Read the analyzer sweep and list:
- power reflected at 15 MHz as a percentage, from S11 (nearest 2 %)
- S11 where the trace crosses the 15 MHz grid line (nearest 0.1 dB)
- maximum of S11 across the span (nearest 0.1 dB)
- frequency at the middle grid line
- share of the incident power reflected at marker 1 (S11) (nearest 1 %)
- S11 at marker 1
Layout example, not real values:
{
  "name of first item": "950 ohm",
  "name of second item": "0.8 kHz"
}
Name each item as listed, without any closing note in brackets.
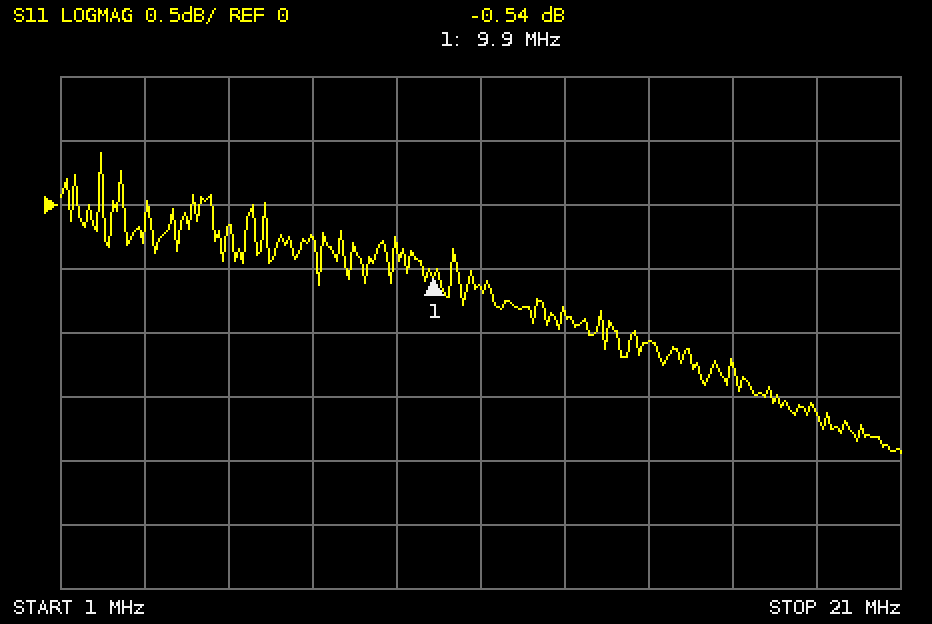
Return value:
{
  "power reflected at 15 MHz as a percentage, from S11": "78 %",
  "S11 where the trace crosses the 15 MHz grid line": "-1.1 dB",
  "maximum of S11 across the span": "0.4 dB",
  "frequency at the middle grid line": "11 MHz",
  "share of the incident power reflected at marker 1 (S11)": "88 %",
  "S11 at marker 1": "-0.54 dB"
}
